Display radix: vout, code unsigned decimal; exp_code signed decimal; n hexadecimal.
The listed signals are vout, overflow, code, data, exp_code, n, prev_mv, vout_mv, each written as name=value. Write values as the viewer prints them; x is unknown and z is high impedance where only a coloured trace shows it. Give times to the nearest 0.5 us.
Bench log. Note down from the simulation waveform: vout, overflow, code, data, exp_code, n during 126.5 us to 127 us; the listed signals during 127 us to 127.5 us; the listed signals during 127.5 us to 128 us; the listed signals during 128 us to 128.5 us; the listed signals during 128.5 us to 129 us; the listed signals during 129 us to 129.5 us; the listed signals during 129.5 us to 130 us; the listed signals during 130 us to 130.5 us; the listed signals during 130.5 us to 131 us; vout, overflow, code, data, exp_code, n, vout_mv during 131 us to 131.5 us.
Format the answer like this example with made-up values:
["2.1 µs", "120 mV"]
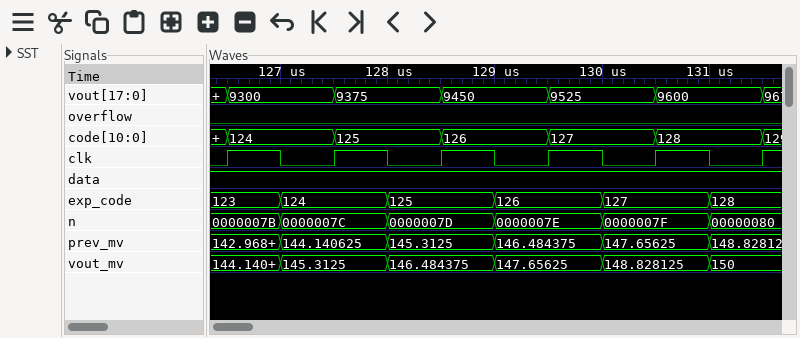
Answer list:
["vout=9300, overflow=0, code=124, data=1, exp_code=123, n=0000007B", "vout=9300, overflow=0, code=124, data=1, exp_code=124, n=0000007C, prev_mv=144.140625, vout_mv=145.3125", "vout=9375, overflow=0, code=125, data=1, exp_code=124, n=0000007C, prev_mv=144.140625, vout_mv=145.3125", "vout=9375, overflow=0, code=125, data=1, exp_code=125, n=0000007D, prev_mv=145.3125, vout_mv=146.484375", "vout=9450, overflow=0, code=126, data=1, exp_code=125, n=0000007D, prev_mv=145.3125, vout_mv=146.484375", "vout=9450, overflow=0, code=126, data=1, exp_code=126, n=0000007E, prev_mv=146.484375, vout_mv=147.65625", "vout=9525, overflow=0, code=127, data=1, exp_code=126, n=0000007E, prev_mv=146.484375, vout_mv=147.65625", "vout=9525, overflow=0, code=127, data=1, exp_code=127, n=0000007F, prev_mv=147.65625, vout_mv=148.828125", "vout=9600, overflow=0, code=128, data=1, exp_code=127, n=0000007F, prev_mv=147.65625, vout_mv=148.828125", "vout=9600, overflow=0, code=128, data=1, exp_code=128, n=00000080, vout_mv=150"]
